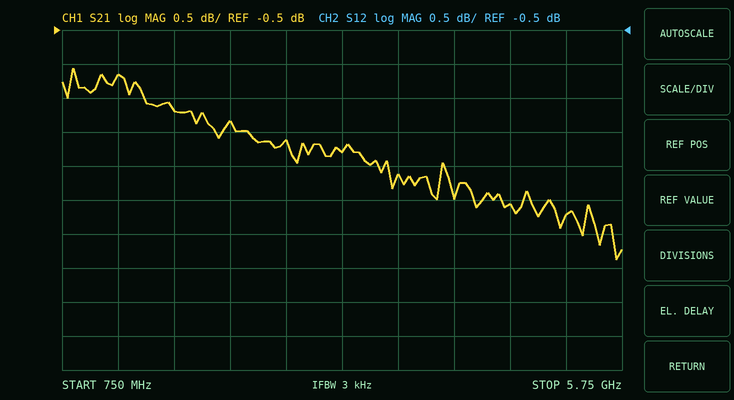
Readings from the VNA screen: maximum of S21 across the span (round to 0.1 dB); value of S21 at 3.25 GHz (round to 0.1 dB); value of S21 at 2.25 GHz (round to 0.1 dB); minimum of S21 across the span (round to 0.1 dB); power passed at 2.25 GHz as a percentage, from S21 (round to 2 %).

-1.1 dB
-2.3 dB
-1.8 dB
-3.9 dB
66 %
